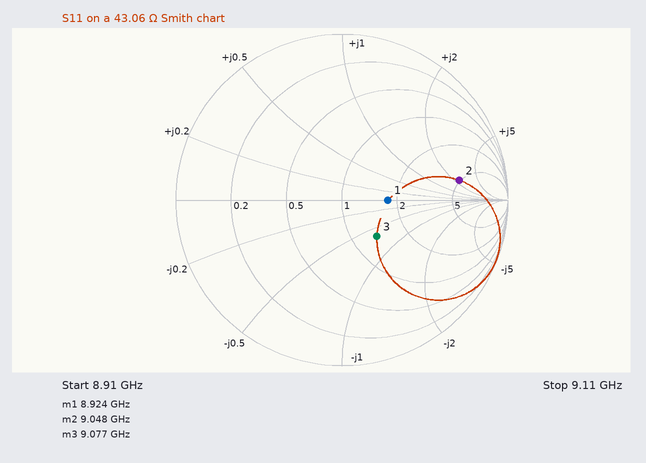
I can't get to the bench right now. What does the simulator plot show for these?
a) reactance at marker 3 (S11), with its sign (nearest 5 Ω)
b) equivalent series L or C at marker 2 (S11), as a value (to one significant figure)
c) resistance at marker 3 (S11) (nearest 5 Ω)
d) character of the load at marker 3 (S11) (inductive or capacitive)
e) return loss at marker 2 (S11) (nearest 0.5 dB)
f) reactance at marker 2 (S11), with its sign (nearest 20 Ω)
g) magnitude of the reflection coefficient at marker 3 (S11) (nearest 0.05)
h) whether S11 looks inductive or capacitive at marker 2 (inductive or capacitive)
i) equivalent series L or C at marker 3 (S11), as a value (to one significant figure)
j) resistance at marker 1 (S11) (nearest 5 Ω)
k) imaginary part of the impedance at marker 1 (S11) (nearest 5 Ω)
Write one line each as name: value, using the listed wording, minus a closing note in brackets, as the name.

reactance at marker 3 (S11), with its sign: -30 Ω
equivalent series L or C at marker 2 (S11), as a value: 2 nH
resistance at marker 3 (S11): 60 Ω
character of the load at marker 3 (S11): capacitive
return loss at marker 2 (S11): 3.0 dB
reactance at marker 2 (S11), with its sign: +100 Ω
magnitude of the reflection coefficient at marker 3 (S11): 0.30
whether S11 looks inductive or capacitive at marker 2: inductive
equivalent series L or C at marker 3 (S11), as a value: 600 fF
resistance at marker 1 (S11): 75 Ω
imaginary part of the impedance at marker 1 (S11): 0 Ω
